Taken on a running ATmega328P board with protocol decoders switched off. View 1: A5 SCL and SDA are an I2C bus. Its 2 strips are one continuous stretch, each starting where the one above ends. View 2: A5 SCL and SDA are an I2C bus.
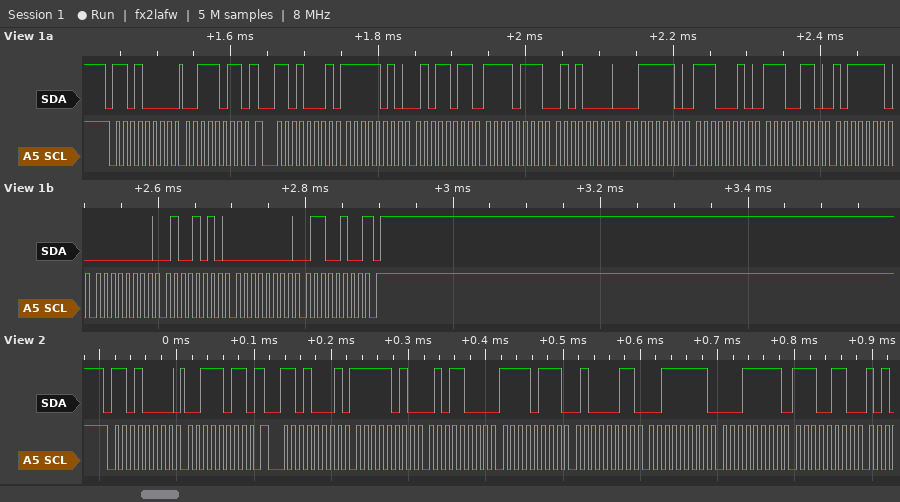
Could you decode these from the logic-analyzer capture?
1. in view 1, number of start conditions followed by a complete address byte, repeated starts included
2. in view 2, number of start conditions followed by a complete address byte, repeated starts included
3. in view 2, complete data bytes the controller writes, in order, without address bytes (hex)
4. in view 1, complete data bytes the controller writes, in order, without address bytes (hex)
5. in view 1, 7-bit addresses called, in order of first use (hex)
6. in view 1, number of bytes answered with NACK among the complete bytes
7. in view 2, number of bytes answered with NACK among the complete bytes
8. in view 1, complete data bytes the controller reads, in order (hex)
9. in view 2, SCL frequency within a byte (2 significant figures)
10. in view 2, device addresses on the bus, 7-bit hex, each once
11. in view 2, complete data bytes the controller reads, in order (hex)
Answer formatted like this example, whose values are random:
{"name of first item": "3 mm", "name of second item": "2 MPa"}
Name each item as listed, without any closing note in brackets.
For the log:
{"in view 1, number of start conditions followed by a complete address byte, repeated starts included": "2", "in view 2, number of start conditions followed by a complete address byte, repeated starts included": "2", "in view 2, complete data bytes the controller writes, in order, without address bytes": "3B", "in view 1, complete data bytes the controller writes, in order, without address bytes": "3B", "in view 1, 7-bit addresses called, in order of first use": "0x68", "in view 1, number of bytes answered with NACK among the complete bytes": "1", "in view 2, number of bytes answered with NACK among the complete bytes": "0", "in view 1, complete data bytes the controller reads, in order": "FA 5B F7 50 3E E2 E6 BE 00 4A 00 64", "in view 2, SCL frequency within a byte": "100 kHz", "in view 2, device addresses on the bus, 7-bit hex, each once": "0x68", "in view 2, complete data bytes the controller reads, in order": "FA 58 F7 43 3F 1F E6"}
